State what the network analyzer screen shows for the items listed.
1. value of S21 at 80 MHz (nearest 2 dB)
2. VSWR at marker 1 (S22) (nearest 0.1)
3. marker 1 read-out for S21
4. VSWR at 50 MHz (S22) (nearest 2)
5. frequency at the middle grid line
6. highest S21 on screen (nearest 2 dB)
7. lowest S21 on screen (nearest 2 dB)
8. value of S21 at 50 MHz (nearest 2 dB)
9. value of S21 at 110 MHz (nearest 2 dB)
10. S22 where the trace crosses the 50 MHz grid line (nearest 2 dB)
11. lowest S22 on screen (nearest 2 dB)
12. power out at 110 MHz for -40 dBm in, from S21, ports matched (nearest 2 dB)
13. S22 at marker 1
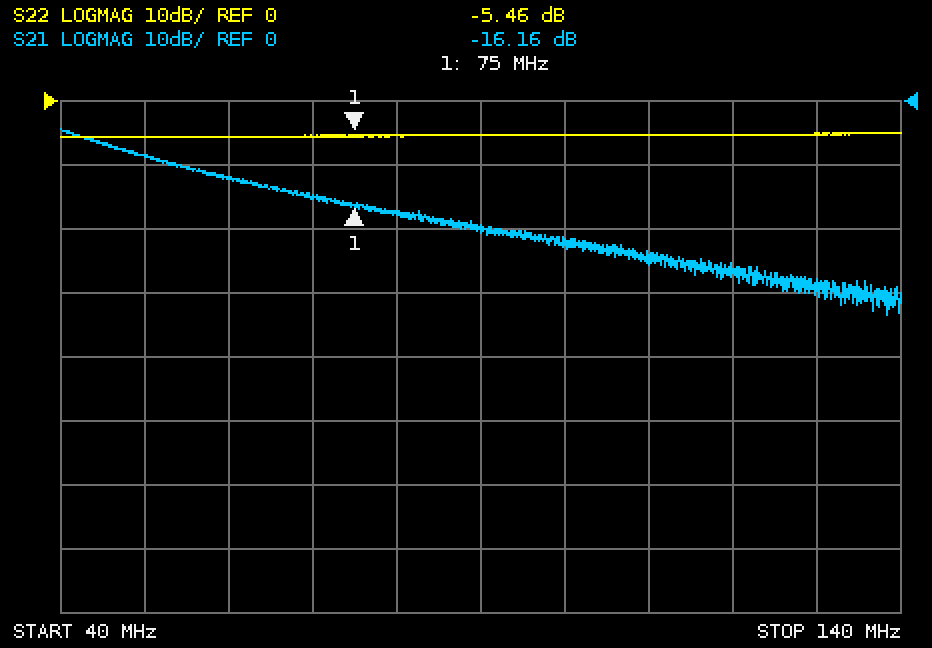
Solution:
-18 dB
3.3
-16.16 dB
4
90 MHz
-4 dB
-34 dB
-8 dB
-24 dB
-6 dB
-6 dB
-64 dBm
-5.46 dB
